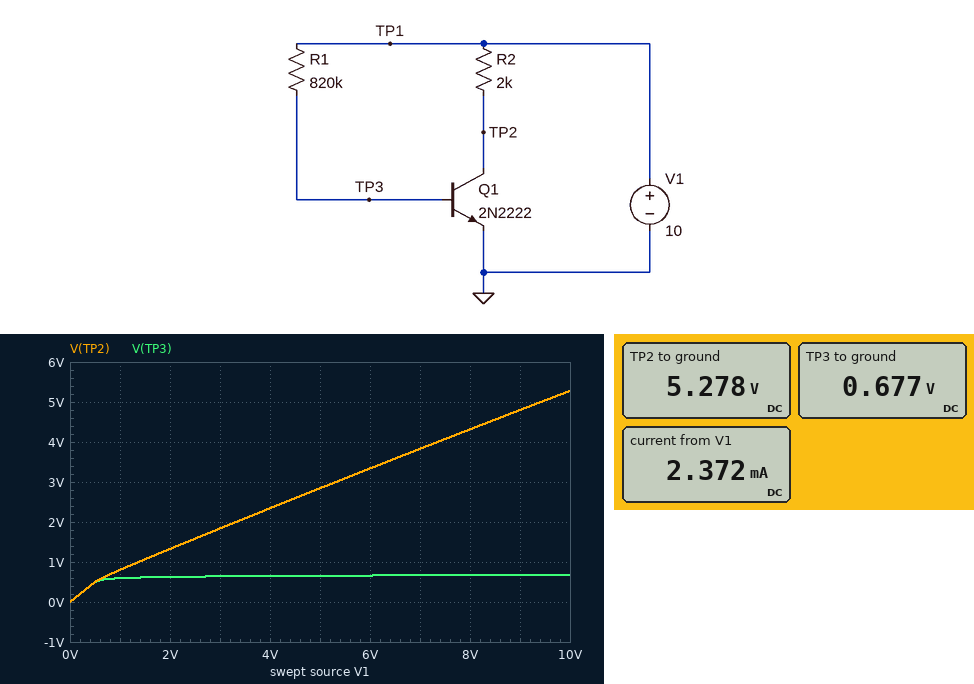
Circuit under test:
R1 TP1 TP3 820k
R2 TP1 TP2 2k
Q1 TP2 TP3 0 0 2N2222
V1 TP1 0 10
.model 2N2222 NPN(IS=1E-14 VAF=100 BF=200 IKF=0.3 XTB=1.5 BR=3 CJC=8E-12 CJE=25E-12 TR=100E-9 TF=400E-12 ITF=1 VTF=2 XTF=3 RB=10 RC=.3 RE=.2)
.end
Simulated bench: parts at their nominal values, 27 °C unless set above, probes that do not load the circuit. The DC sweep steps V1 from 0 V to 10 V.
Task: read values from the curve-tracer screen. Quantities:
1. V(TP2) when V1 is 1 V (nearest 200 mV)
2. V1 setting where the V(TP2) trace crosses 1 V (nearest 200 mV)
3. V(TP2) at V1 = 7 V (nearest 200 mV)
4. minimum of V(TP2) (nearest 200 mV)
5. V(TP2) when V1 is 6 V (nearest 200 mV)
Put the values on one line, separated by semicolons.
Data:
800 mV; 1.4 V; 3.8 V; 0 V; 3.4 V
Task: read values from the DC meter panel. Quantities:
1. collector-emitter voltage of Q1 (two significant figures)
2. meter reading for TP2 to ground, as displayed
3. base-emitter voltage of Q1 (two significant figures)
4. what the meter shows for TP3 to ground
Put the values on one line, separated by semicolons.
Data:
5.3 V; 5.278 V; 680 mV; 0.677 V
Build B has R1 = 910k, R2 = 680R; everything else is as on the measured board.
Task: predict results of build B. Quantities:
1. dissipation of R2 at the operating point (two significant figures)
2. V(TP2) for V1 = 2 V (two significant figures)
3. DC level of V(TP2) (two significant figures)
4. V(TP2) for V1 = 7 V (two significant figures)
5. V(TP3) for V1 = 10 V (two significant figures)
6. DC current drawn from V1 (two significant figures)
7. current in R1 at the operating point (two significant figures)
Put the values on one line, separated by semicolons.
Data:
3.3 mW; 1.8 V; 8.5 V; 6.0 V; 670 mV; 2.2 mA; 10 µA
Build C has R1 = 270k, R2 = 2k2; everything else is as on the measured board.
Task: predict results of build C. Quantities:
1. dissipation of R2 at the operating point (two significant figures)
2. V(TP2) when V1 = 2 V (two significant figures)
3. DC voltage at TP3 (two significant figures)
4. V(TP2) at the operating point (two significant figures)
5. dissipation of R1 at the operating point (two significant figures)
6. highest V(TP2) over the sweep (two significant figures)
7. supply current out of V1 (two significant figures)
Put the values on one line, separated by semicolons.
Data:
44 mW; 150 mV; 700 mV; 130 mV; 320 µW; 540 mV; 4.5 mA
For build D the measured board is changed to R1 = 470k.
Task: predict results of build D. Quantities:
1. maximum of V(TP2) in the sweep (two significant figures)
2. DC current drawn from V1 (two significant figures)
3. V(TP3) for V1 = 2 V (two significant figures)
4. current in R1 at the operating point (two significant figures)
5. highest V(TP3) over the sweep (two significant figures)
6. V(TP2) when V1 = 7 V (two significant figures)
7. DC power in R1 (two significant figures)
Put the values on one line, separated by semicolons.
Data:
2.1 V; 4.0 mA; 640 mV; 20 µA; 690 mV; 1.6 V; 180 µW
